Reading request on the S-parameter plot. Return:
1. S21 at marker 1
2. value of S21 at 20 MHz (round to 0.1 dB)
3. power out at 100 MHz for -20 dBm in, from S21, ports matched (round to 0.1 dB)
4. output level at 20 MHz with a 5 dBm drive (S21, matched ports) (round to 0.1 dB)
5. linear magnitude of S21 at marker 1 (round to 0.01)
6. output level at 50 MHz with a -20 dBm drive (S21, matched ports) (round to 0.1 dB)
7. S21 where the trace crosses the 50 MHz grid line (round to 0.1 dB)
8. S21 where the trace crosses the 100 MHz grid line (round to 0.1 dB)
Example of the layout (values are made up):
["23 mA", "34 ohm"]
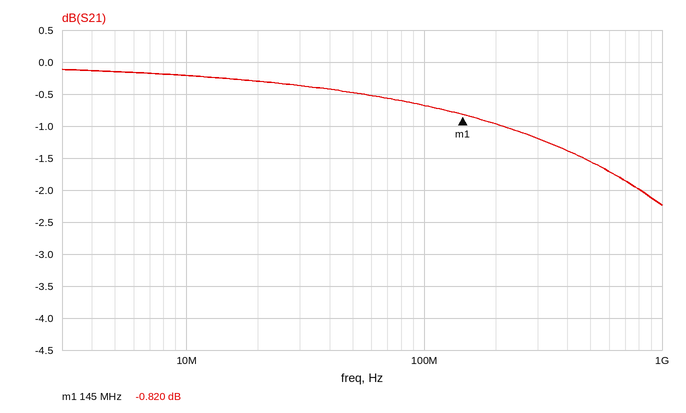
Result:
["-0.820 dB", "-0.3 dB", "-20.7 dBm", "4.7 dBm", "0.91", "-20.5 dBm", "-0.5 dB", "-0.7 dB"]
